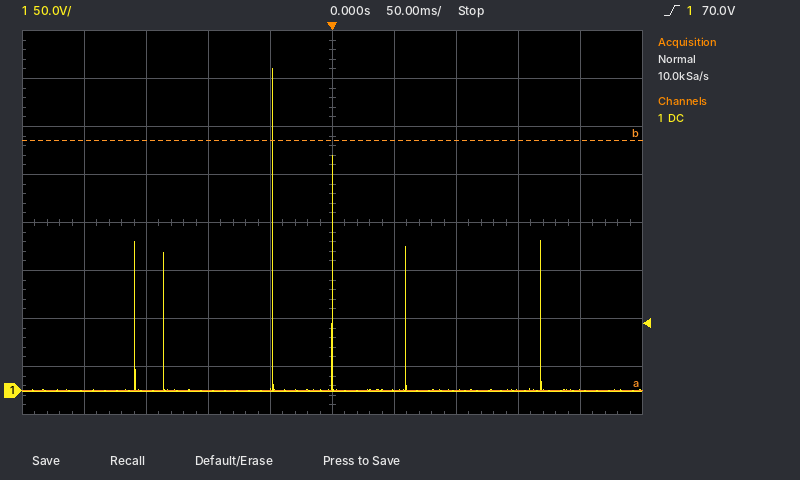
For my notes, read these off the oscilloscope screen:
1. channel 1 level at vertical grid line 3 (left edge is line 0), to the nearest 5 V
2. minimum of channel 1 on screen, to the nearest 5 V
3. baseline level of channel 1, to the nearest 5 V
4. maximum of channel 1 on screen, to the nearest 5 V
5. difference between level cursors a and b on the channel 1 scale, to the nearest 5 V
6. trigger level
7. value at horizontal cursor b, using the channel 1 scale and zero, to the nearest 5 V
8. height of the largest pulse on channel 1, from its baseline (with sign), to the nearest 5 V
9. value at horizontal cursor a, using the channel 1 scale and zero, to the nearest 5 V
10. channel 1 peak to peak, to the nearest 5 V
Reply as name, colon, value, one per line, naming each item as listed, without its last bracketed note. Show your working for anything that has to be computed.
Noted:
channel 1 level at vertical grid line 3 (left edge is line 0), to the nearest 5 V: 0 V
minimum of channel 1 on screen, to the nearest 5 V: 0 V
baseline level of channel 1, to the nearest 5 V: 0 V
maximum of channel 1 on screen, to the nearest 5 V: 335 V
difference between level cursors a and b on the channel 1 scale, to the nearest 5 V: 260 V
trigger level: 70.0 V
value at horizontal cursor b, using the channel 1 scale and zero, to the nearest 5 V: 260 V
height of the largest pulse on channel 1, from its baseline (with sign), to the nearest 5 V: 335 V − (0 V) = +335 V
value at horizontal cursor a, using the channel 1 scale and zero, to the nearest 5 V: 0 V
channel 1 peak to peak, to the nearest 5 V: 335 V − (0 V) = 335 V
